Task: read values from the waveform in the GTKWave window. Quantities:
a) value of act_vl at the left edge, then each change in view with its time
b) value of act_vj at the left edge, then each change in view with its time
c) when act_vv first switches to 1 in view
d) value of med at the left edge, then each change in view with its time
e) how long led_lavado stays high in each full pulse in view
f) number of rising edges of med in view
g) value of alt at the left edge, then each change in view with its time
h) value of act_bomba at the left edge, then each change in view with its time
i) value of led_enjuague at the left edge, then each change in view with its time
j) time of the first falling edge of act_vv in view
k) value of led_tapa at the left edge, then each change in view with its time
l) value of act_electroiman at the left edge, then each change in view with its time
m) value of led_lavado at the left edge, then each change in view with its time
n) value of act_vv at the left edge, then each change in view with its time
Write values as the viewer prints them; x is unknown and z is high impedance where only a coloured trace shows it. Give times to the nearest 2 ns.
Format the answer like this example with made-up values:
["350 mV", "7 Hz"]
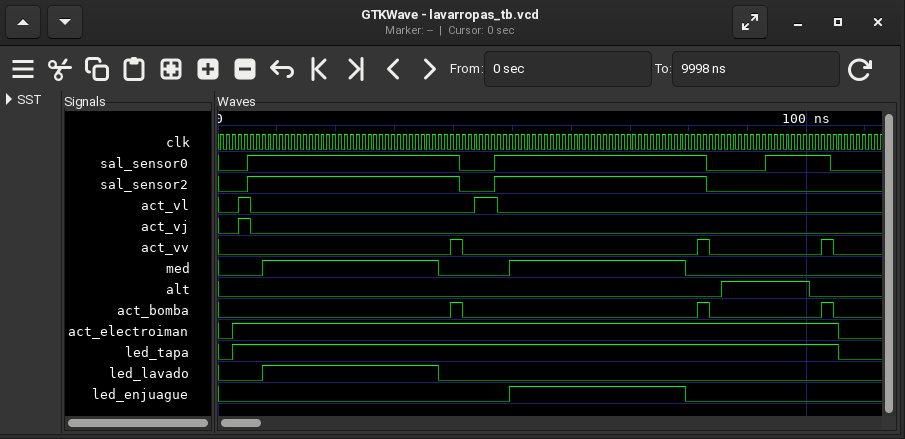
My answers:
["0, 1 at 4 ns, 0 at 6 ns, 1 at 44 ns, 0 at 48 ns", "0, 1 at 4 ns, 0 at 6 ns", "40 ns", "0, 1 at 8 ns, 0 at 38 ns, 1 at 50 ns, 0 at 80 ns", "30 ns", "2", "0, 1 at 86 ns, 0 at 100 ns", "0, 1 at 40 ns, 0 at 42 ns, 1 at 82 ns, 0 at 84 ns, 1 at 102 ns, 0 at 104 ns", "0, 1 at 50 ns, 0 at 80 ns", "42 ns", "0, 1 at 2 ns, 0 at 106 ns", "0, 1 at 2 ns, 0 at 106 ns", "0, 1 at 8 ns, 0 at 38 ns", "0, 1 at 40 ns, 0 at 42 ns, 1 at 82 ns, 0 at 84 ns, 1 at 102 ns, 0 at 104 ns"]
